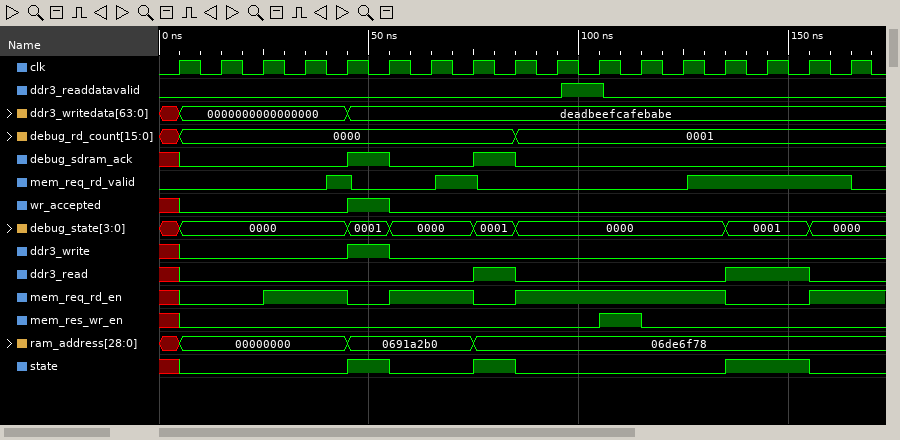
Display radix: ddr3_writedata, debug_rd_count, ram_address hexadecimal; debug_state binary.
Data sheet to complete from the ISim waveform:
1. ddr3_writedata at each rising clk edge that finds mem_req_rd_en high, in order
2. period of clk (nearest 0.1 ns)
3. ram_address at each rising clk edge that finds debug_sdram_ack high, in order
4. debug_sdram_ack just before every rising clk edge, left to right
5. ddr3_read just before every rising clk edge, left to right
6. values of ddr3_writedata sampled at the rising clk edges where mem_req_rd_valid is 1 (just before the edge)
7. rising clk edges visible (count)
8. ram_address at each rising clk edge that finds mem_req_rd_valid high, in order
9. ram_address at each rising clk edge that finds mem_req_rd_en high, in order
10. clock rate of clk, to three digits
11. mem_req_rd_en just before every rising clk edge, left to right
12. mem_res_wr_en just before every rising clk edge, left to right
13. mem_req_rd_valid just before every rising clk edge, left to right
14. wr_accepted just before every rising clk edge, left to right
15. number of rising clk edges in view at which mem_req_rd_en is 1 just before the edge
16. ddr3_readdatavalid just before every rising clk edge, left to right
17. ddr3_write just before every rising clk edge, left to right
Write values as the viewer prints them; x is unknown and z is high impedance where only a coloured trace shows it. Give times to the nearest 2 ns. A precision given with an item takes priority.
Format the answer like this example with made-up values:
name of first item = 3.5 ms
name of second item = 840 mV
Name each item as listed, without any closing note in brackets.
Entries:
ddr3_writedata at each rising clk edge that finds mem_req_rd_en high, in order = 0000000000000000, 0000000000000000, deadbeefcafebabe, deadbeefcafebabe, deadbeefcafebabe, deadbeefcafebabe, deadbeefcafebabe, deadbeefcafebabe, deadbeefcafebabe, deadbeefcafebabe
period of clk = 10 ns
ram_address at each rising clk edge that finds debug_sdram_ack high, in order = 0691a2b0, 06de6f78
debug_sdram_ack just before every rising clk edge, left to right = x 0 0 0 0 1 0 0 1 0 0 0 0 0 0 0 0
ddr3_read just before every rising clk edge, left to right = x 0 0 0 0 0 0 0 1 0 0 0 0 0 1 1 0
values of ddr3_writedata sampled at the rising clk edges where mem_req_rd_valid is 1 = 0000000000000000, deadbeefcafebabe, deadbeefcafebabe, deadbeefcafebabe, deadbeefcafebabe, deadbeefcafebabe
rising clk edges visible = 17
ram_address at each rising clk edge that finds mem_req_rd_valid high, in order = 00000000, 0691a2b0, 06de6f78, 06de6f78, 06de6f78, 06de6f78
ram_address at each rising clk edge that finds mem_req_rd_en high, in order = 00000000, 00000000, 0691a2b0, 0691a2b0, 06de6f78, 06de6f78, 06de6f78, 06de6f78, 06de6f78, 06de6f78
clock rate of clk, to three digits = 100 MHz
mem_req_rd_en just before every rising clk edge, left to right = x 0 0 1 1 0 1 1 0 1 1 1 1 1 0 0 1
mem_res_wr_en just before every rising clk edge, left to right = x 0 0 0 0 0 0 0 0 0 0 1 0 0 0 0 0
mem_req_rd_valid just before every rising clk edge, left to right = 0 0 0 0 1 0 0 1 0 0 0 0 0 1 1 1 1
wr_accepted just before every rising clk edge, left to right = x 0 0 0 0 1 0 0 0 0 0 0 0 0 0 0 0
number of rising clk edges in view at which mem_req_rd_en is 1 just before the edge = 10
ddr3_readdatavalid just before every rising clk edge, left to right = 0 0 0 0 0 0 0 0 0 0 1 0 0 0 0 0 0
ddr3_write just before every rising clk edge, left to right = x 0 0 0 0 1 0 0 0 0 0 0 0 0 0 0 0
